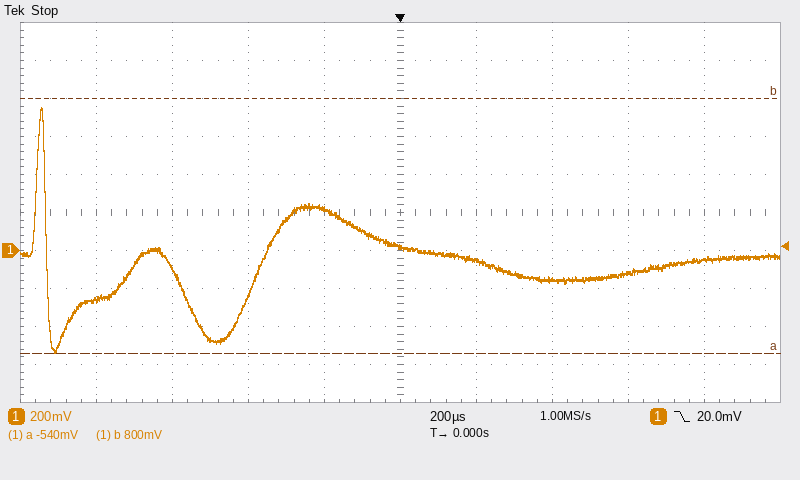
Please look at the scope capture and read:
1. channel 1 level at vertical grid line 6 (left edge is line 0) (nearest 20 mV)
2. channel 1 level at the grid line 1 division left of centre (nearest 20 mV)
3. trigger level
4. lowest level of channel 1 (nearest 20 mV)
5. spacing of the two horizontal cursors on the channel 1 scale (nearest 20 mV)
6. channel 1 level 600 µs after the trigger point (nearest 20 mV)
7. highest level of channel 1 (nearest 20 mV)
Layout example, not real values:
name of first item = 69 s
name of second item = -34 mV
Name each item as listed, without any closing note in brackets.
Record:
channel 1 level at vertical grid line 6 (left edge is line 0) = -60 mV
channel 1 level at the grid line 1 division left of centre = 220 mV
trigger level = 20.0 mV
lowest level of channel 1 = -540 mV
spacing of the two horizontal cursors on the channel 1 scale = 1.34 V
channel 1 level 600 µs after the trigger point = -120 mV
highest level of channel 1 = 760 mV
